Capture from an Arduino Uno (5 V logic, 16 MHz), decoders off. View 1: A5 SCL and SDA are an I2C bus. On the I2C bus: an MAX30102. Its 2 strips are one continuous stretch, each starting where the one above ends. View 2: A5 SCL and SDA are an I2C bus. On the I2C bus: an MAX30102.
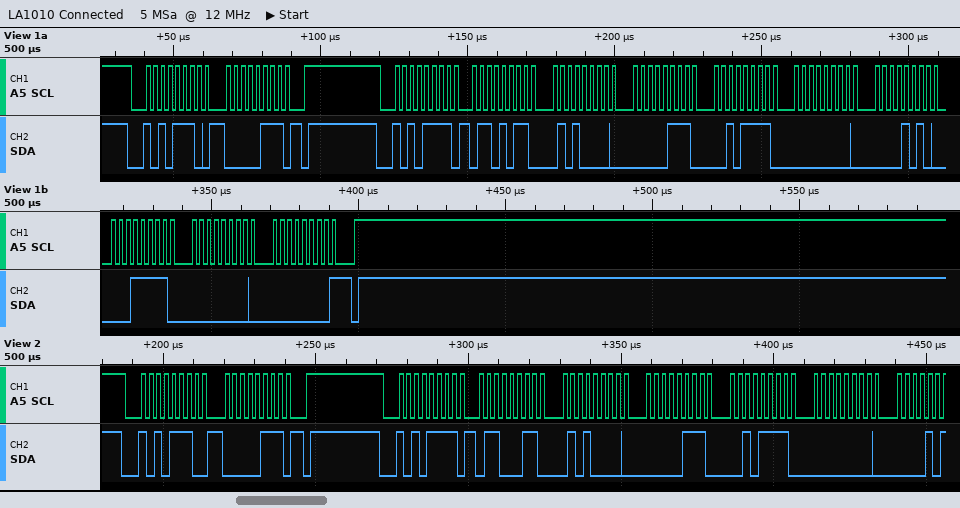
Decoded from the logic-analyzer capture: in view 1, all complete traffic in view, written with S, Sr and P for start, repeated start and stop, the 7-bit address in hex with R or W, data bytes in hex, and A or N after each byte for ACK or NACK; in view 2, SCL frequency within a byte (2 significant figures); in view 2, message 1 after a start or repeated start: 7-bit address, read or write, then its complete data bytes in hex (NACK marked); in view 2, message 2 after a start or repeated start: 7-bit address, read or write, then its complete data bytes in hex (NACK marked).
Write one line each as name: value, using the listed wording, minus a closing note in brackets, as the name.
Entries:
in view 1, all complete traffic in view, written with S, Sr and P for start, repeated start and stop, the 7-bit address in hex with R or W, data bytes in hex, and A or N after each byte for ACK or NACK: S 57W A 07 A P S 57R A 6B A 50 A 07 A 2F A 00 A 0A A 1F A 00 A 00 N P
in view 2, SCL frequency within a byte: 400 kHz
in view 2, message 1 after a start or repeated start: 7-bit address, read or write, then its complete data bytes in hex: 0x57 write: 07
in view 2, message 2 after a start or repeated start: 7-bit address, read or write, then its complete data bytes in hex: 0x57 read: 63 50 07 2F 00
